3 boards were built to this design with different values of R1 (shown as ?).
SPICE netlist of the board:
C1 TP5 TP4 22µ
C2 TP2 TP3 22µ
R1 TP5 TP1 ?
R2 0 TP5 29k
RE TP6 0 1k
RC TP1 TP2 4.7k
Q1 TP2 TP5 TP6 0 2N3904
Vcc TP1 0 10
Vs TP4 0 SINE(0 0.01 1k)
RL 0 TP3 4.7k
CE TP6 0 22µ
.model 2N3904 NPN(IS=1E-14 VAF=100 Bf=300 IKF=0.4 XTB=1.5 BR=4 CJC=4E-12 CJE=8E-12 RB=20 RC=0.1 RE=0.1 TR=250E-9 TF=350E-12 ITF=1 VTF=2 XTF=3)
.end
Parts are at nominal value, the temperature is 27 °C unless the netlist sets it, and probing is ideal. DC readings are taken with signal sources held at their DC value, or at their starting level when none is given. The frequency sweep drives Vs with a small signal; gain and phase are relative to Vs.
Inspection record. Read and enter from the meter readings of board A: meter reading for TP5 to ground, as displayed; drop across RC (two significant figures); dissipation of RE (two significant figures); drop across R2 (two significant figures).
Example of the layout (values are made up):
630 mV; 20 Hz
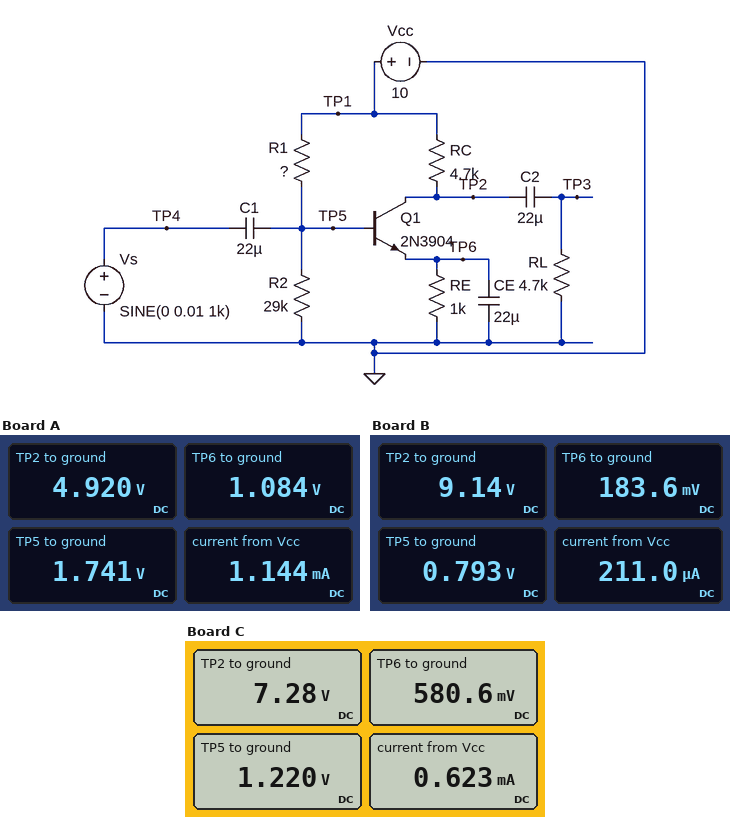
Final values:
1.741 V; 5.1 V; 1.2 mW; 1.7 V
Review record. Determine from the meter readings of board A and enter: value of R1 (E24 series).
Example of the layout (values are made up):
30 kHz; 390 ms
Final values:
130 kΩ
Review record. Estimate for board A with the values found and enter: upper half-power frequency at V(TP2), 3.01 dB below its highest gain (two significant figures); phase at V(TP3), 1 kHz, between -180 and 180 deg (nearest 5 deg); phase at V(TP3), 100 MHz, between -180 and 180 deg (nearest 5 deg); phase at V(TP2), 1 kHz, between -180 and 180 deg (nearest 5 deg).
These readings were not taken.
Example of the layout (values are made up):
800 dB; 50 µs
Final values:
16 MHz; -165 deg; 85 deg; -165 deg
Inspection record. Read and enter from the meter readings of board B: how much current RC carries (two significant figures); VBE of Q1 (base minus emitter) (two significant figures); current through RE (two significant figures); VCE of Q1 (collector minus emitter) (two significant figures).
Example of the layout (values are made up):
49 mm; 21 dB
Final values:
180 µA; 610 mV; 180 µA; 9.0 V
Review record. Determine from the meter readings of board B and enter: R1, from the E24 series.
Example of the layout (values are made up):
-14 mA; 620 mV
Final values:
330 kΩ
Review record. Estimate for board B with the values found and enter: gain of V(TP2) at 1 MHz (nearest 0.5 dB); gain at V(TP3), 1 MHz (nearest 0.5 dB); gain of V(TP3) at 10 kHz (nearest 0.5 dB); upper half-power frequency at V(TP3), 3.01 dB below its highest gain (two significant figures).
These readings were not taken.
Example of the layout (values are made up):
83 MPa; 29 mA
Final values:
24.5 dB; 24.5 dB; 24.5 dB; 33 MHz
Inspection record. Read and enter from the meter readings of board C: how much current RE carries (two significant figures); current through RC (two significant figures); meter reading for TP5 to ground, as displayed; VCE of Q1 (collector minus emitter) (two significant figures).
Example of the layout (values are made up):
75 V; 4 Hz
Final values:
580 µA; 580 µA; 1.220 V; 6.7 V
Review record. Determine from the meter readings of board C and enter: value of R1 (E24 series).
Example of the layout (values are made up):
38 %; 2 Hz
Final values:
200 kΩ
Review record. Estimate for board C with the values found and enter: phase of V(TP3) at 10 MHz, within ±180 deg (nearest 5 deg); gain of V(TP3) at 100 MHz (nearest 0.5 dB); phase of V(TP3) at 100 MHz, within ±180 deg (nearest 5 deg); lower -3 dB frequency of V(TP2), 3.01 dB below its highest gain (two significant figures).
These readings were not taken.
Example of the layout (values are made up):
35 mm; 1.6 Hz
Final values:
155 deg; 21.5 dB; 90 deg; 170 Hz
